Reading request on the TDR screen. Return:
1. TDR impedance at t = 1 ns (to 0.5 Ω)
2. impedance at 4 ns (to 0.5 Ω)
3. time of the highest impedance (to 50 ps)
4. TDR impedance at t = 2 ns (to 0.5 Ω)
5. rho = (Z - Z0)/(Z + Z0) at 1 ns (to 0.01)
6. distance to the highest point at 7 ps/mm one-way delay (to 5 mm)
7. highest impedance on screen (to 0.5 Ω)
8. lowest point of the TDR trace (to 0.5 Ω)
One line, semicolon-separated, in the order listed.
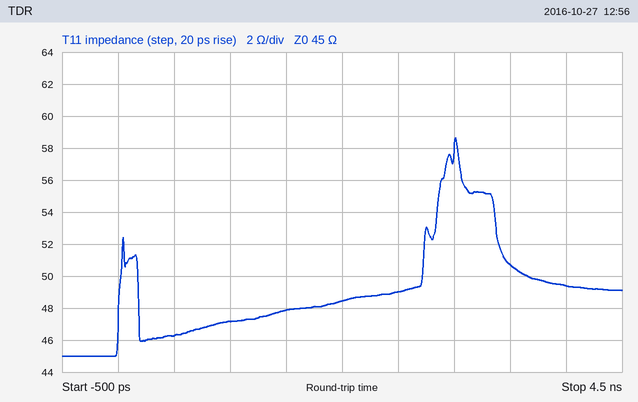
47.0 Ω; 49.5 Ω; 3.00 ns; 48.5 Ω; +0.02; 215 mm; 58.5 Ω; 45.0 Ω
